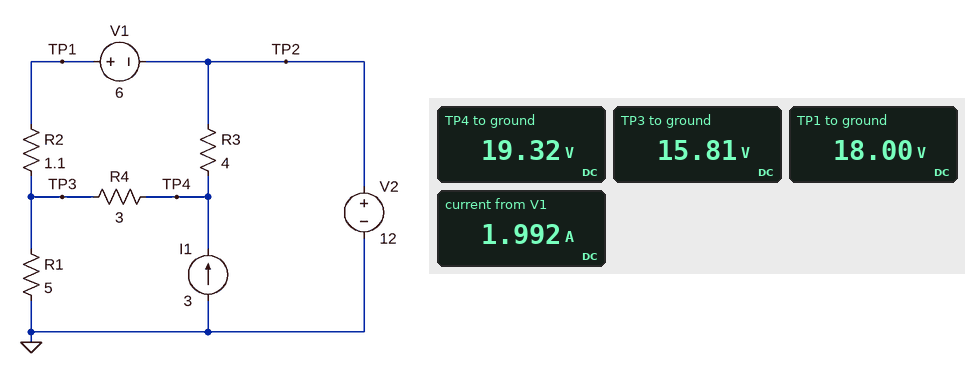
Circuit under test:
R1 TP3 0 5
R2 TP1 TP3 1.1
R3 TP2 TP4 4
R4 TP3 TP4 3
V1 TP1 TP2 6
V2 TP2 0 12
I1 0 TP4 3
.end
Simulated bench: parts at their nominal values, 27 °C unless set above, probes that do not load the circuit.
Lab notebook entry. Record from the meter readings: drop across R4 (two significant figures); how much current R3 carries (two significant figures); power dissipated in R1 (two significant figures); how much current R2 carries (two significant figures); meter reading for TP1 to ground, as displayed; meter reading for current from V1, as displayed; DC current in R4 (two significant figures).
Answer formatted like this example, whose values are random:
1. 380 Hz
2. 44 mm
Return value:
1. 3.5 V
2. 1.8 A
3. 50 W
4. 2.0 A
5. 18.00 V
6. 1.992 A
7. 1.2 A
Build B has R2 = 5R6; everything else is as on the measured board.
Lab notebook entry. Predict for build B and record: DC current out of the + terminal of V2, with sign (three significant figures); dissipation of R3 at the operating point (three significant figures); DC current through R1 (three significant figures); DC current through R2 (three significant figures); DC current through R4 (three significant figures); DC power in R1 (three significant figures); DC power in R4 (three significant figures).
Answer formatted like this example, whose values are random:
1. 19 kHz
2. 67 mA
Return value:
1. -452 mA
2. 7.74 W
3. 2.55 A
4. 939 mA
5. 1.61 A
6. 32.5 W
7. 7.76 W
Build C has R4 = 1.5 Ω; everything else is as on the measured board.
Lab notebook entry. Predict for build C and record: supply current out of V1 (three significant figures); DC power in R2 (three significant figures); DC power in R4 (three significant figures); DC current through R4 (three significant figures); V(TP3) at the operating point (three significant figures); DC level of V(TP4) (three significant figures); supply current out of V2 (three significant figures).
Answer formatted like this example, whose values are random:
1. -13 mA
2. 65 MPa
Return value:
1. 1.77 A
2. 3.43 W
3. 3.13 W
4. 1.44 A
5. 16.1 V
6. 18.2 V
7. 211 mA
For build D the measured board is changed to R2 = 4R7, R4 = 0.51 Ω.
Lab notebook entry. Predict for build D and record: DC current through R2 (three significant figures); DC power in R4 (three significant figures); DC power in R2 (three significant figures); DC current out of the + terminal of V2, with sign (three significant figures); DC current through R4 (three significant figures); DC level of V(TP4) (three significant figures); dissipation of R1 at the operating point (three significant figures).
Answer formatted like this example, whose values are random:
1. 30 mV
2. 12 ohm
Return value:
1. 761 mA
2. 2.30 W
3. 2.72 W
4. -115 mA
5. 2.12 A
6. 15.5 V
7. 41.6 W
